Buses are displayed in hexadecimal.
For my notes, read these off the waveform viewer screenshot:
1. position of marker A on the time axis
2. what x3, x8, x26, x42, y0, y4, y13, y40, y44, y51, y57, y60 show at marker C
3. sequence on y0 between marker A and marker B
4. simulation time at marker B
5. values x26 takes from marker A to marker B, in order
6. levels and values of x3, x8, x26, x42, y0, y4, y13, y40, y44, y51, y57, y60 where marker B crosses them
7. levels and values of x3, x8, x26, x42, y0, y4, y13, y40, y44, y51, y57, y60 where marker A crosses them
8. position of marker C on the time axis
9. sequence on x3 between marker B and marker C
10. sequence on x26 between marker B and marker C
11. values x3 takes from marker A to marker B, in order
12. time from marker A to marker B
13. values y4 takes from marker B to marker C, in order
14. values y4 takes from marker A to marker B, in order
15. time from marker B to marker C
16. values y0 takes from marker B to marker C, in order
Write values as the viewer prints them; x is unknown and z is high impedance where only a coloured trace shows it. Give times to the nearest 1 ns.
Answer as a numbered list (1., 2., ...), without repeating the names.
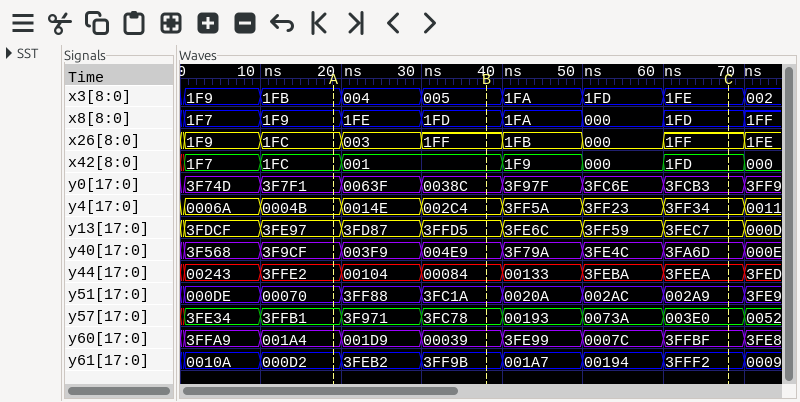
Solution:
1. 19 ns
2. x3=1FE, x8=1FD, x26=1FF, x42=1FD, y0=3FCB3, y4=3FF34, y13=3FEC7, y40=3FA6D, y44=3FEEA, y51=002A9, y57=003E0, y60=3FFBF
3. 3F7F1, 0063F, 0038C
4. 38 ns
5. 1FC, 003, 1FF
6. x3=005, x8=1FD, x26=1FF, x42=001, y0=0038C, y4=002C4, y13=3FFD5, y40=004E9, y44=00084, y51=3FC1A, y57=3FC78, y60=00039
7. x3=1FB, x8=1F9, x26=1FC, x42=1FC, y0=3F7F1, y4=0004B, y13=3FE97, y40=3F9CF, y44=3FFE2, y51=00070, y57=3FFB1, y60=001A4
8. 68 ns
9. 005, 1FA, 1FD, 1FE
10. 1FF, 1FB, 000, 1FF
11. 1FB, 004, 005
12. 19 ns
13. 002C4, 3FF5A, 3FF23, 3FF34
14. 0004B, 0014E, 002C4
15. 30 ns
16. 0038C, 3F97F, 3FC6E, 3FCB3
